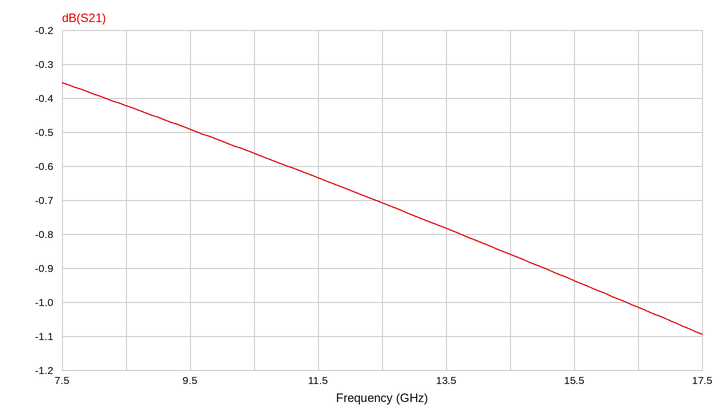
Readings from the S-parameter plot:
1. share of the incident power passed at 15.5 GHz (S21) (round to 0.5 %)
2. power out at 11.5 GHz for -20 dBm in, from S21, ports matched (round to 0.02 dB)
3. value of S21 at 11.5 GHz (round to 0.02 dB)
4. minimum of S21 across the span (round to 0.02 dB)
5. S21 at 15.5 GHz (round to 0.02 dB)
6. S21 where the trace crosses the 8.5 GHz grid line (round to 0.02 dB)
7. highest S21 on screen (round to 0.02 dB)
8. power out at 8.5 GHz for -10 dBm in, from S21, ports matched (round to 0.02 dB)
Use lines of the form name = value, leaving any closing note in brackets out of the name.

share of the incident power passed at 15.5 GHz (S21) = 80.5 %
power out at 11.5 GHz for -20 dBm in, from S21, ports matched = -20.64 dBm
value of S21 at 11.5 GHz = -0.64 dB
minimum of S21 across the span = -1.10 dB
S21 at 15.5 GHz = -0.94 dB
S21 where the trace crosses the 8.5 GHz grid line = -0.42 dB
highest S21 on screen = -0.36 dB
power out at 8.5 GHz for -10 dBm in, from S21, ports matched = -10.42 dBm
